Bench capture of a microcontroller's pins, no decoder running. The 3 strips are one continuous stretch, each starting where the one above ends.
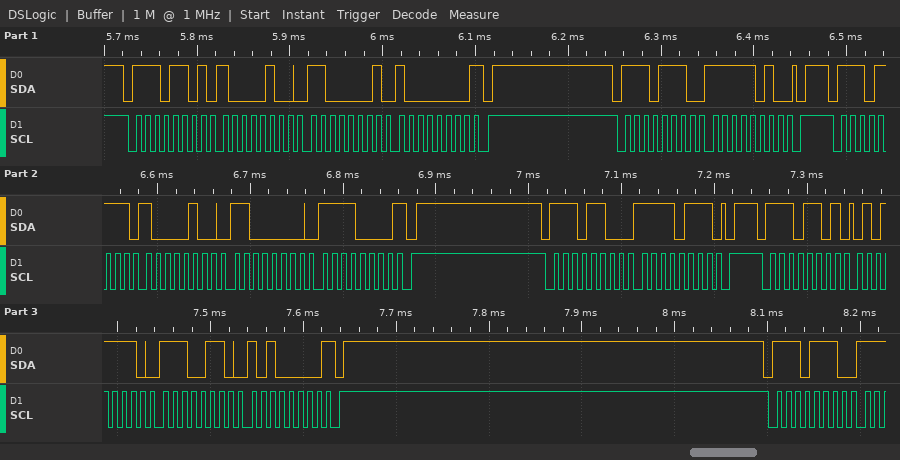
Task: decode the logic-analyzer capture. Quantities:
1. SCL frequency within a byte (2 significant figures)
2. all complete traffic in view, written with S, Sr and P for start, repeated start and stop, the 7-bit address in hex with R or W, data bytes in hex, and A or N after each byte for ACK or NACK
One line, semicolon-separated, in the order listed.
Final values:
100 kHz; S 76R A 84 A C1 A 80 N P S 77W A FA A P S 77R A 84 A C0 A F0 N P S 76W A F7 A P S 76R A 5E A E6 A A0 N P S 77W A
